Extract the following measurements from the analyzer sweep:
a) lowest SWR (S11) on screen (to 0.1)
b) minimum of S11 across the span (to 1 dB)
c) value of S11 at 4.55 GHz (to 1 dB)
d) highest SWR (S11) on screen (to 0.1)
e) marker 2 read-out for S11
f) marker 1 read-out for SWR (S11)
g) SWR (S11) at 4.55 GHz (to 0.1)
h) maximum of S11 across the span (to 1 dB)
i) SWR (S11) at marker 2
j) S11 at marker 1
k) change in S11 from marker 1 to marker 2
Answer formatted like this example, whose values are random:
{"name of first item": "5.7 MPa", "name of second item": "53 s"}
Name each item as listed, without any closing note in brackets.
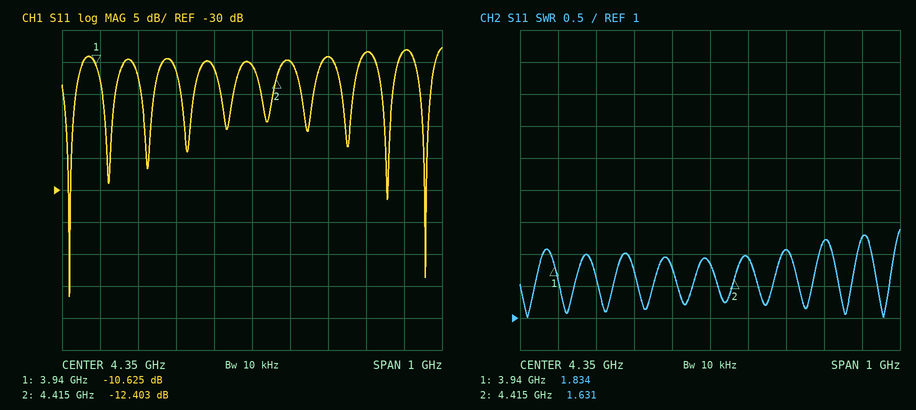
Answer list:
{"lowest SWR (S11) on screen": "1.0", "minimum of S11 across the span": "-47 dB", "value of S11 at 4.55 GHz": "-9 dB", "highest SWR (S11) on screen": "2.4", "marker 2 read-out for S11": "-12.403 dB", "marker 1 read-out for SWR": "1.834", "SWR (S11) at 4.55 GHz": "2.1", "maximum of S11 across the span": "-8 dB", "SWR (S11) at marker 2": "1.631", "S11 at marker 1": "-10.625 dB", "change in S11 from marker 1 to marker 2": "-1.778 dB"}
